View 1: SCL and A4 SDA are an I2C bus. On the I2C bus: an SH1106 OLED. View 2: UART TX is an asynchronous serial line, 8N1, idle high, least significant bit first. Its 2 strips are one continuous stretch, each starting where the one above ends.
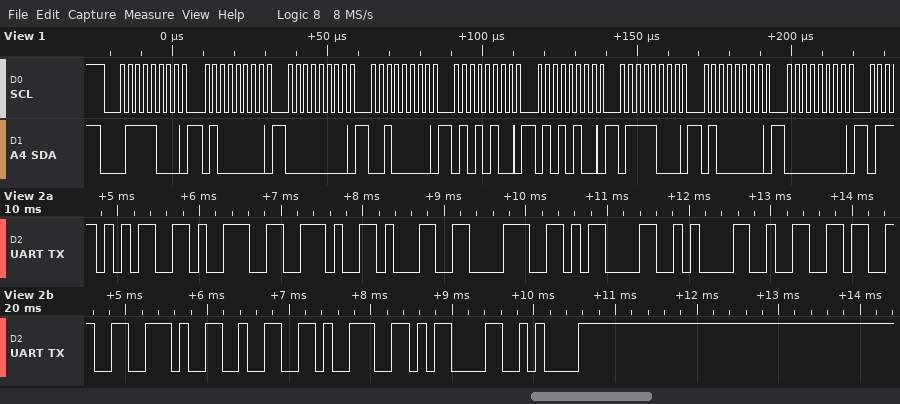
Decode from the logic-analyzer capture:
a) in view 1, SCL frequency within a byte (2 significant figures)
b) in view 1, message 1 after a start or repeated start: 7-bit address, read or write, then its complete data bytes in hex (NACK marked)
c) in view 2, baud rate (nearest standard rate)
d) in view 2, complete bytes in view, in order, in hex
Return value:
400 kHz
0x3C write: 40 00 20 54 54 78 40 00
9600 baud
35 39 2E 31 38 0D 0A 32 33 2E 32 39 0D 0A
